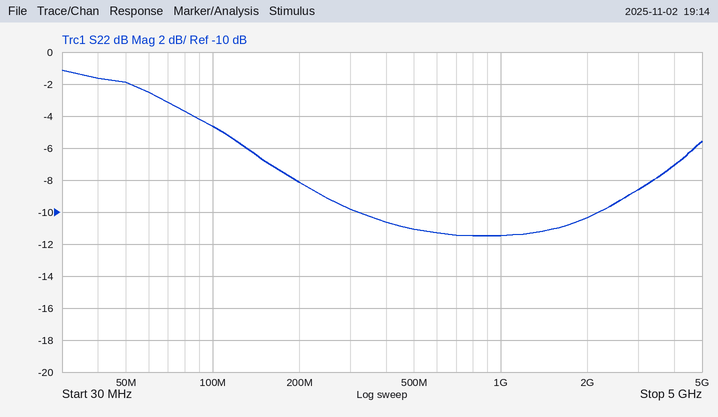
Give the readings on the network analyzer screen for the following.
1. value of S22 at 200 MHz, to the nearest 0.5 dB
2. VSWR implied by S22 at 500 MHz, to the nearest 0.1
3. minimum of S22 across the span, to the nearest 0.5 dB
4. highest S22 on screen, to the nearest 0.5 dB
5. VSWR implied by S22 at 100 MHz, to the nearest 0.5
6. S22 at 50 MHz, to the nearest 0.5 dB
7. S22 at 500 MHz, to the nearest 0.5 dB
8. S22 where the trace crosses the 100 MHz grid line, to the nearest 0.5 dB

-8.0 dB
1.8
-11.5 dB
-1.0 dB
4.0
-2.0 dB
-11.0 dB
-4.5 dB
